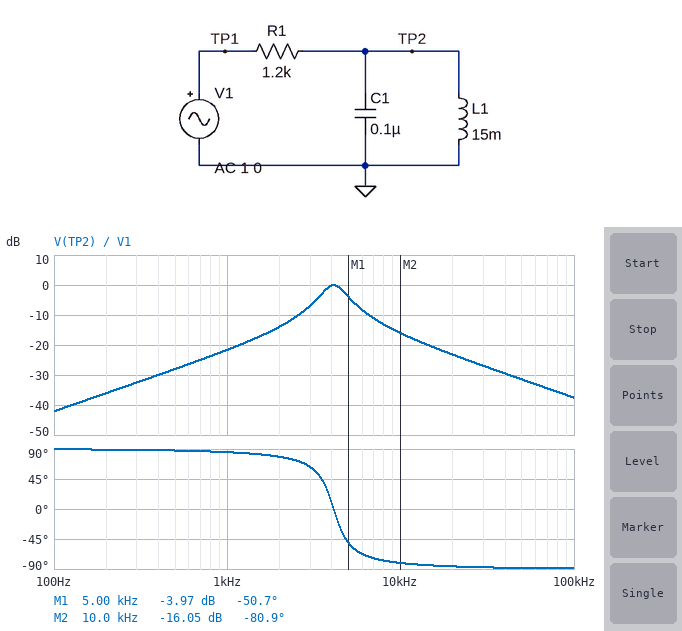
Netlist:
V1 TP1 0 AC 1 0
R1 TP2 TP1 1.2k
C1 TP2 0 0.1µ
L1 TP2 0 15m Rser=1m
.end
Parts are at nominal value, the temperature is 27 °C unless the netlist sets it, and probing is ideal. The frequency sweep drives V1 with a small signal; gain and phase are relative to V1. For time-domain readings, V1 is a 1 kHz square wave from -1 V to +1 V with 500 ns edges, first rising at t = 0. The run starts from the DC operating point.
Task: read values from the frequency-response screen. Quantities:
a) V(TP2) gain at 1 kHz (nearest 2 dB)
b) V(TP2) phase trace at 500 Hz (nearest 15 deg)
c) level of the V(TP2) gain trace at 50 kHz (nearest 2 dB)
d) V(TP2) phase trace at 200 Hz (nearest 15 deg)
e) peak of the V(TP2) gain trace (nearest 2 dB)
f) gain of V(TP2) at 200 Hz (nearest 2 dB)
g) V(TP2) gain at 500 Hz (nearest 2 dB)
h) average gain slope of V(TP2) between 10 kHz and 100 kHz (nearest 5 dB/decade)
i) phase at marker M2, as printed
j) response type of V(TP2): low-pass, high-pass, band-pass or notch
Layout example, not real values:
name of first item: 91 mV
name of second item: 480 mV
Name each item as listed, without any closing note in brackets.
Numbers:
V(TP2) gain at 1 kHz: -22 dB
V(TP2) phase trace at 500 Hz: 90 deg
level of the V(TP2) gain trace at 50 kHz: -32 dB
V(TP2) phase trace at 200 Hz: 90 deg
peak of the V(TP2) gain trace: 0 dB
gain of V(TP2) at 200 Hz: -36 dB
V(TP2) gain at 500 Hz: -28 dB
average gain slope of V(TP2) between 10 kHz and 100 kHz: -20 dB/decade
phase at marker M2, as printed: -80.9 deg
response type of V(TP2): low-pass, high-pass, band-pass or notch: band-pass
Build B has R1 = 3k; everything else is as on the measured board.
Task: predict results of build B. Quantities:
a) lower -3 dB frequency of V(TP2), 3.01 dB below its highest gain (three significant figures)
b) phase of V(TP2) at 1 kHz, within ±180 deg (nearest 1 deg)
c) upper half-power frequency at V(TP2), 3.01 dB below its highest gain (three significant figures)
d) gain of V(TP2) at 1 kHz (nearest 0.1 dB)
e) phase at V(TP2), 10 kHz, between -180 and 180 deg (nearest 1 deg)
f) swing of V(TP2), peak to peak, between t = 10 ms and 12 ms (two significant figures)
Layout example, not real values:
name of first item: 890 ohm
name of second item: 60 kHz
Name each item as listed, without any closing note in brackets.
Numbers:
lower -3 dB frequency of V(TP2), 3.01 dB below its highest gain: 3.85 kHz
phase of V(TP2) at 1 kHz, within ±180 deg: 88 deg
upper half-power frequency at V(TP2), 3.01 dB below its highest gain: 4.38 kHz
gain of V(TP2) at 1 kHz: -29.5 dB
phase at V(TP2), 10 kHz, between -180 and 180 deg: -86 deg
swing of V(TP2), peak to peak, between t = 10 ms and 12 ms: 330 mV
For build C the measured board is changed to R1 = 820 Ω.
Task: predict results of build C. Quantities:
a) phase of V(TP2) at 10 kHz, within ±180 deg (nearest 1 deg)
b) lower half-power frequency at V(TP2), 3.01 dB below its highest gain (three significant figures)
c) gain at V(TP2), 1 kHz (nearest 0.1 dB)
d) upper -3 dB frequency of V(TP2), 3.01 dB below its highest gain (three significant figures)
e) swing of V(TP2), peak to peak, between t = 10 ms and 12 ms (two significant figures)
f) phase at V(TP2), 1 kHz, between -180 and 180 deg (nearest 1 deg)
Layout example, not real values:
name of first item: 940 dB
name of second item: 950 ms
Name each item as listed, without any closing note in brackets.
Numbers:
phase of V(TP2) at 10 kHz, within ±180 deg: -77 deg
lower half-power frequency at V(TP2), 3.01 dB below its highest gain: 3.25 kHz
gain at V(TP2), 1 kHz: -18.3 dB
upper -3 dB frequency of V(TP2), 3.01 dB below its highest gain: 5.19 kHz
swing of V(TP2), peak to peak, between t = 10 ms and 12 ms: 1.3 V
phase at V(TP2), 1 kHz, between -180 and 180 deg: 83 deg
